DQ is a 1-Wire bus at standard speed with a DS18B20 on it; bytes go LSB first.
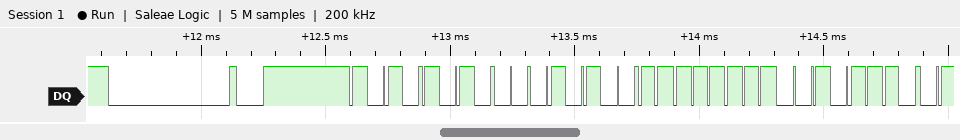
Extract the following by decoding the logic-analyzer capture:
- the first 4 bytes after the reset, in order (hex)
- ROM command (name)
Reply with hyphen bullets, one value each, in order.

- 55 28 FF 74
- Match ROM
